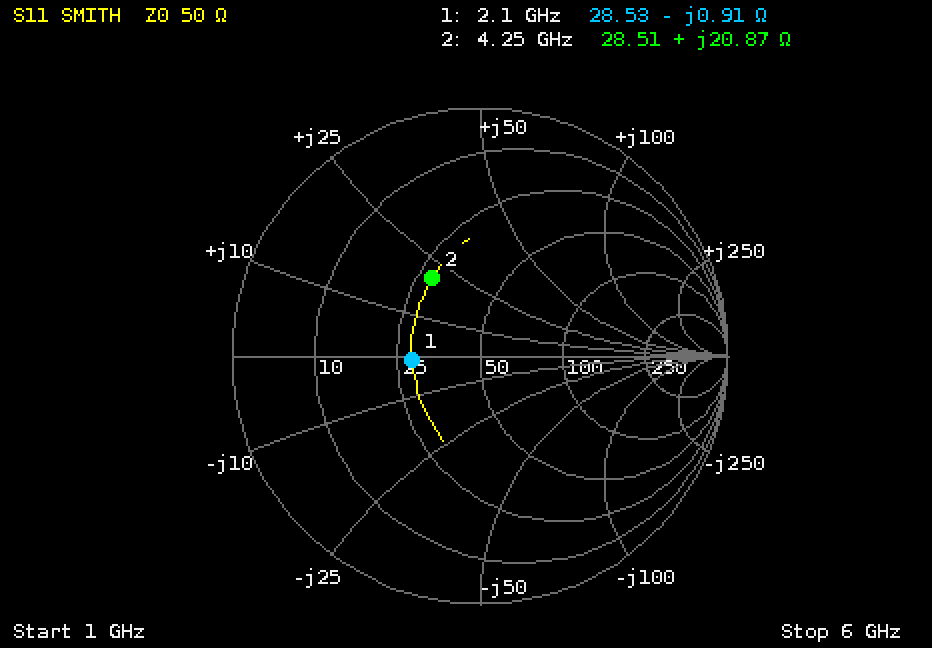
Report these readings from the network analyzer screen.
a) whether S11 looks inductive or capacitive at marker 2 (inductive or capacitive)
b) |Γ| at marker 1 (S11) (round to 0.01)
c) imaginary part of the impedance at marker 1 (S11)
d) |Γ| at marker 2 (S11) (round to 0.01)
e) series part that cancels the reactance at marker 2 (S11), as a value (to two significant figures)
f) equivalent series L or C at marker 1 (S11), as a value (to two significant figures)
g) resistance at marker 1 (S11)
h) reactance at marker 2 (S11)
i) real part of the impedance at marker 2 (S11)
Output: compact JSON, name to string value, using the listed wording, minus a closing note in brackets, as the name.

{"whether S11 looks inductive or capacitive at marker 2": "inductive", "|Γ| at marker 1 (S11)": "0.27", "imaginary part of the impedance at marker 1": "-0.91 Ω", "|Γ| at marker 2 (S11)": "0.37", "series part that cancels the reactance at marker 2 (S11), as a value": "1.8 pF", "equivalent series L or C at marker 1 (S11), as a value": "83 pF", "resistance at marker 1": "28.53 Ω", "reactance at marker 2": "+20.87 Ω", "real part of the impedance at marker 2": "28.51 Ω"}
